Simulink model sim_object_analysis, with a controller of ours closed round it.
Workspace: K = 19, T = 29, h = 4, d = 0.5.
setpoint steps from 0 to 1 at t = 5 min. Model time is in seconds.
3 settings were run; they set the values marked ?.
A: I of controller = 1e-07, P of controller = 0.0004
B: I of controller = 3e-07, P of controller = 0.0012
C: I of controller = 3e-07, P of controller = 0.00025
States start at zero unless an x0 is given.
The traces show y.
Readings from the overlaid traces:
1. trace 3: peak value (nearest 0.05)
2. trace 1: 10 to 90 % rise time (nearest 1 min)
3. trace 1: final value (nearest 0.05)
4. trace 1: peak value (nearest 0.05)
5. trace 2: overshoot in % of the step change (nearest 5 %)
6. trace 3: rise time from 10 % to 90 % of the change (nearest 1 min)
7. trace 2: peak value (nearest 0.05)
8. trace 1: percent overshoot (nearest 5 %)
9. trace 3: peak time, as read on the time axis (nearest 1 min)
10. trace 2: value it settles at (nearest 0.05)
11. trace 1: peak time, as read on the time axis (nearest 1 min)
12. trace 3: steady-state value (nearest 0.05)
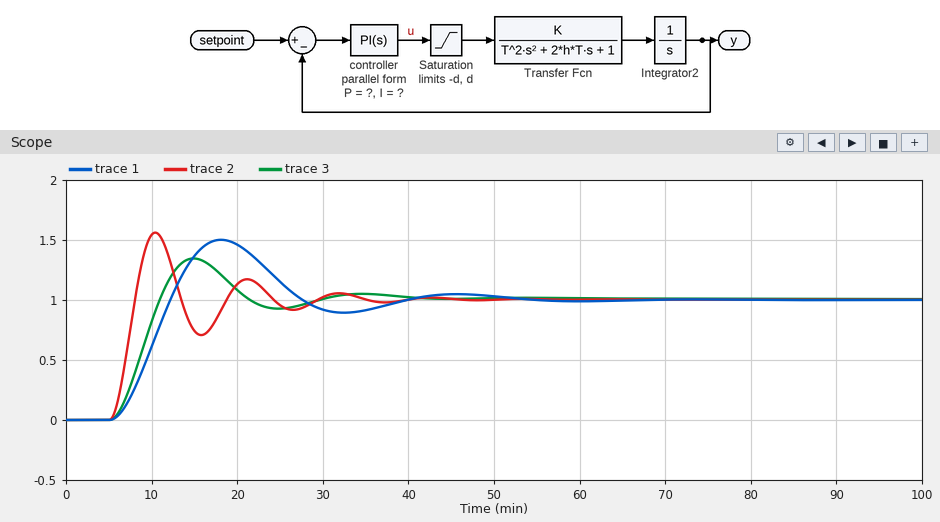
1.35
5 min
1.00
1.50
55 %
4 min
1.55
50 %
15 min
1.00
18 min
1.00
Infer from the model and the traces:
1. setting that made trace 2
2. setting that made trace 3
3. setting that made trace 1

B
A
C
